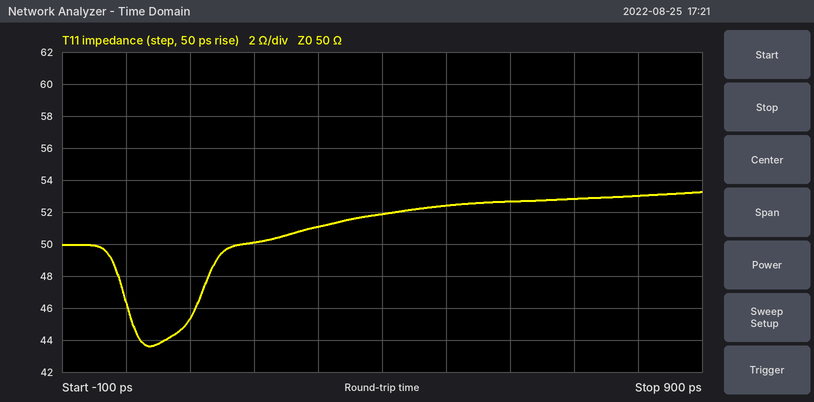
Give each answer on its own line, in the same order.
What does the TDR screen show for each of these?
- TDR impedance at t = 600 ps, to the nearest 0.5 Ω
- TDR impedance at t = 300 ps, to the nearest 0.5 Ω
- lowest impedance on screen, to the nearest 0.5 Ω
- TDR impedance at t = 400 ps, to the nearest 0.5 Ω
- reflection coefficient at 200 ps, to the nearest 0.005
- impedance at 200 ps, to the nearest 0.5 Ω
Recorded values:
52.5 Ω
51.0 Ω
43.5 Ω
52.0 Ω
0.000
50.0 Ω
